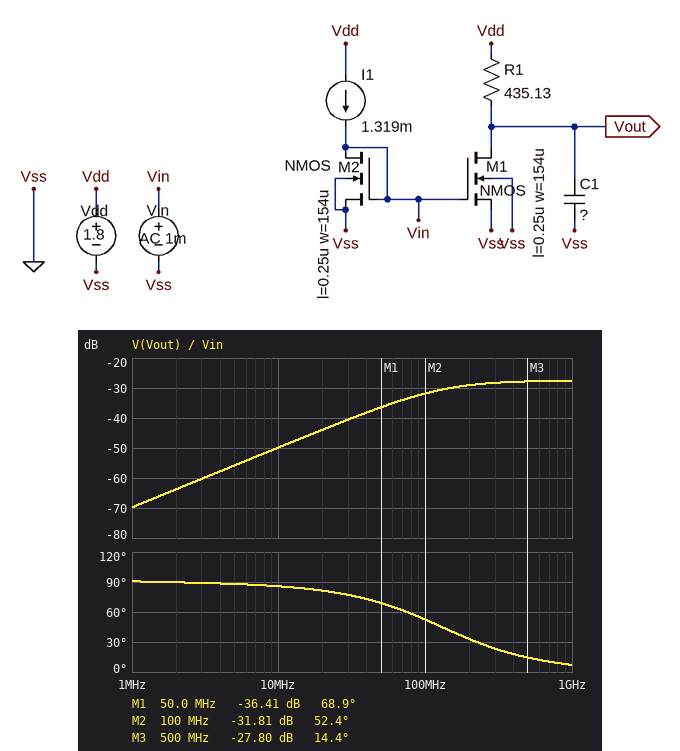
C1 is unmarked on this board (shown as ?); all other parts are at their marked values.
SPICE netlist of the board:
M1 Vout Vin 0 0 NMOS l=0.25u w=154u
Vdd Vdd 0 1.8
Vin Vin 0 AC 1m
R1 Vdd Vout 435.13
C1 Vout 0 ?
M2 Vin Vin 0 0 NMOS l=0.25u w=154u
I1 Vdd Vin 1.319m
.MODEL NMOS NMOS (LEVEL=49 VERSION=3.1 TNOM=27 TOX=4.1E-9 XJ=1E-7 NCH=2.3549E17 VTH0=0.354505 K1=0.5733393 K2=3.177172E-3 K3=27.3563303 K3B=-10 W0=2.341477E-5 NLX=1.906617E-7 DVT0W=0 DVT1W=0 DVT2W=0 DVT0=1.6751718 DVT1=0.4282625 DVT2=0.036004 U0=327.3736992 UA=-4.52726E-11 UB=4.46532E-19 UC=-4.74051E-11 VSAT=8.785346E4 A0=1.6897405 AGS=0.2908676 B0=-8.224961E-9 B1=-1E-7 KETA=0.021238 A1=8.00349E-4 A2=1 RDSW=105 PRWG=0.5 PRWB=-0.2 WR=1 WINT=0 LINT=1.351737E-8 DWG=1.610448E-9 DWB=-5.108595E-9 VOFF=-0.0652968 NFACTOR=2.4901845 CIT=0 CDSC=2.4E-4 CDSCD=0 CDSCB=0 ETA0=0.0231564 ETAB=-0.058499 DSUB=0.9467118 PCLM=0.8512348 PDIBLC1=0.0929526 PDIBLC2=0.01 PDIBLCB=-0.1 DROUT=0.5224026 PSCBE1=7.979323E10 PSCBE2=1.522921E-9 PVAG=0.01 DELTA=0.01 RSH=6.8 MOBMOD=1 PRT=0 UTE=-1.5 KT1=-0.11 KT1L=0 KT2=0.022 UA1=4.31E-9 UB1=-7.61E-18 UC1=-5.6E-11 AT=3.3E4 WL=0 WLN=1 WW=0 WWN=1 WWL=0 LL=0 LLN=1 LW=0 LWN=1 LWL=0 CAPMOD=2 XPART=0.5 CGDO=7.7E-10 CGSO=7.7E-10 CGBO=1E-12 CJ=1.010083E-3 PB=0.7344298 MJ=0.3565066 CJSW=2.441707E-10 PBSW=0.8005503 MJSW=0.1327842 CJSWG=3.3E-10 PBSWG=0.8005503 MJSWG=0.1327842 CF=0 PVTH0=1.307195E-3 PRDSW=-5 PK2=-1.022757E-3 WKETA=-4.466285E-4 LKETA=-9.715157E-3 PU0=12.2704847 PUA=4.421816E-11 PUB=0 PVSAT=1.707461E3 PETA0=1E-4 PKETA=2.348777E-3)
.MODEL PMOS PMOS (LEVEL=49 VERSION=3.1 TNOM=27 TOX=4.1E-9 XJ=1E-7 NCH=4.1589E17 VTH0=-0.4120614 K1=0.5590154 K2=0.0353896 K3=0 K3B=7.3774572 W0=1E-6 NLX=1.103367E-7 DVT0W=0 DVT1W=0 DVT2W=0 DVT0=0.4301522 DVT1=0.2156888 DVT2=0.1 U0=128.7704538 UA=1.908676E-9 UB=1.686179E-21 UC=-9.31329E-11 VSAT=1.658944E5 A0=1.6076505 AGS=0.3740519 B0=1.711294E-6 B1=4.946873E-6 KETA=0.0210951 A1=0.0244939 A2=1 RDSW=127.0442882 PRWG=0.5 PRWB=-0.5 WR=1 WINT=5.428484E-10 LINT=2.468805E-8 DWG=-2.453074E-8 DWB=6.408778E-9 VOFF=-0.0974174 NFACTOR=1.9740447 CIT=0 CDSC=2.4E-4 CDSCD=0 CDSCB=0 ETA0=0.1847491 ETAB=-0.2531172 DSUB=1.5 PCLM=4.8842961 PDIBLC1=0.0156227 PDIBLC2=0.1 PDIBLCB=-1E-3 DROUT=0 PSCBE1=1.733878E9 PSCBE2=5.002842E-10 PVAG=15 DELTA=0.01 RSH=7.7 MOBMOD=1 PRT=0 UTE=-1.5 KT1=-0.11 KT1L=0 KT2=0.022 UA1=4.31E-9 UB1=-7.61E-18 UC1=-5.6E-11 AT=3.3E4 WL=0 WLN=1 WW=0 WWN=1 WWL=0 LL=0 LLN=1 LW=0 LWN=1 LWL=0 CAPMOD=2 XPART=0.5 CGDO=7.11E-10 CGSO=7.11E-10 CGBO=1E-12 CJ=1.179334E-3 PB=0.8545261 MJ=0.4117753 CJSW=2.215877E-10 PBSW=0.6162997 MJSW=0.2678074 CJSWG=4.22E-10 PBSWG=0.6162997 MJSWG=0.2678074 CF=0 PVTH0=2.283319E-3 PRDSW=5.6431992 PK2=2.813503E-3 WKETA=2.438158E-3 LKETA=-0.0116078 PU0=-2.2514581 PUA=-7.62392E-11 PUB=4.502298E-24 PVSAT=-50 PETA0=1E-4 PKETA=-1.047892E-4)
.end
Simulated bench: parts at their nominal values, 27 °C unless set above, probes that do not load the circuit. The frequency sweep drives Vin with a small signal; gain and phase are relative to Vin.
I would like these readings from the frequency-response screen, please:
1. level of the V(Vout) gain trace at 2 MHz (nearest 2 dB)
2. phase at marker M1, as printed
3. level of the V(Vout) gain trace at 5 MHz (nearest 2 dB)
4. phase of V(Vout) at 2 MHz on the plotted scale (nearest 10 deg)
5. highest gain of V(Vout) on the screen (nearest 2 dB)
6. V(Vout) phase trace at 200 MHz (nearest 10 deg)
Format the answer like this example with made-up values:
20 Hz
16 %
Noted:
-64 dB
68.9 deg
-56 dB
90 deg
-28 dB
30 deg
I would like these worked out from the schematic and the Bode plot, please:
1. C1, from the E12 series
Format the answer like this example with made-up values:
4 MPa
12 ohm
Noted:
2.7 pF
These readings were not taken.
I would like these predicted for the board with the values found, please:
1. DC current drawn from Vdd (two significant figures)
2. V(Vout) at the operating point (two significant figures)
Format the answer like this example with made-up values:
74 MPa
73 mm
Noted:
1.3 mA
1.8 V
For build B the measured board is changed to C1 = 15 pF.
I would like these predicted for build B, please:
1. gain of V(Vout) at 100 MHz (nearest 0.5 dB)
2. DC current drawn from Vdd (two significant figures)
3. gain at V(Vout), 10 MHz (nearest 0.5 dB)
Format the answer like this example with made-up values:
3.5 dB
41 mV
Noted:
-42.5 dB
1.3 mA
-50.5 dB
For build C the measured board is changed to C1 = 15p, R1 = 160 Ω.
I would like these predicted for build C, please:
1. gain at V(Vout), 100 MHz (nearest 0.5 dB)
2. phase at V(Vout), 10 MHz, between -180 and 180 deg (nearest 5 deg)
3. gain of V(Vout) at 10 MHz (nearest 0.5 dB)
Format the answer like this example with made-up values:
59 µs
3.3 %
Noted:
-43.5 dB
80 deg
-58.5 dB
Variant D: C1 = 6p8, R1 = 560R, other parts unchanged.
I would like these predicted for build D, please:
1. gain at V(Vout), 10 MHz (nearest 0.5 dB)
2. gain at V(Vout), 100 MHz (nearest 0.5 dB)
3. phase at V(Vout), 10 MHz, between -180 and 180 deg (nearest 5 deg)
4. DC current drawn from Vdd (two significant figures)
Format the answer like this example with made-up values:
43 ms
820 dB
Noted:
-48.0 dB
-36.0 dB
75 deg
1.3 mA
